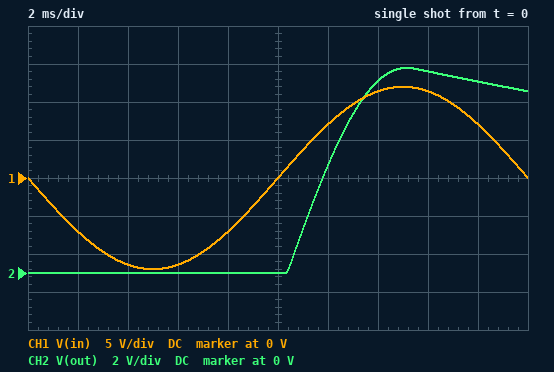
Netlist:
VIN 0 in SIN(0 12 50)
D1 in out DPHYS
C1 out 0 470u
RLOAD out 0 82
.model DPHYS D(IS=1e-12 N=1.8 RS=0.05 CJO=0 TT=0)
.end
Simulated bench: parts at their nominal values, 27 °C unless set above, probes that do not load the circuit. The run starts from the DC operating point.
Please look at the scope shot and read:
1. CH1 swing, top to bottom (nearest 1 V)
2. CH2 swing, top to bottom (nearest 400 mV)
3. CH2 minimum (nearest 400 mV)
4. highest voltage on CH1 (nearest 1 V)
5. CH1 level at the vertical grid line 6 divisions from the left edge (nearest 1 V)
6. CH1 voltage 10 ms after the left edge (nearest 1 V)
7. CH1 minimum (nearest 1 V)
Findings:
24 V
10.8 V
0 V
12 V
7 V
0 V
-12 V
